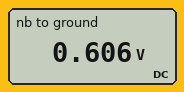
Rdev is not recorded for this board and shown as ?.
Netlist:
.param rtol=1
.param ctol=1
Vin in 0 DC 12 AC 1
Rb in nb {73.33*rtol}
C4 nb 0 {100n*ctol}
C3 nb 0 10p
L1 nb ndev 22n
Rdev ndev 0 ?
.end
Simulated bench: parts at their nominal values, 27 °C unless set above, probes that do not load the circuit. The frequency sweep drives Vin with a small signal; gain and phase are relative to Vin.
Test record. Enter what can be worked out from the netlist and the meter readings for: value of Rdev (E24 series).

3.9 Ω
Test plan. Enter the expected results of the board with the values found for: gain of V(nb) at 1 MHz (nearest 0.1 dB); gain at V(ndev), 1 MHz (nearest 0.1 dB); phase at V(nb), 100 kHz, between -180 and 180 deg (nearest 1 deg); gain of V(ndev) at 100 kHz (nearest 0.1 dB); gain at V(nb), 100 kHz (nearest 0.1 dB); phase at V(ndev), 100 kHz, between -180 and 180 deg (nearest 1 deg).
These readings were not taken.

-33.9 dB
-33.9 dB
-13 deg
-26.2 dB
-26.2 dB
-13 deg
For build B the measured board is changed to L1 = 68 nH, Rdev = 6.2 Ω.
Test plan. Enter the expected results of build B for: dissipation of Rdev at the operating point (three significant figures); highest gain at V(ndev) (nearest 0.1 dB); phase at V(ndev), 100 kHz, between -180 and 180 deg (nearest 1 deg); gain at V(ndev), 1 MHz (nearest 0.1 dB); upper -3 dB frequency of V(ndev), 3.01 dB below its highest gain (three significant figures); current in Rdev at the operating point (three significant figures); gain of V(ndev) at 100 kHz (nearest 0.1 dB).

141 mW
-22.2 dB
-20 deg
-33.5 dB
283 kHz
151 mA
-22.7 dB
